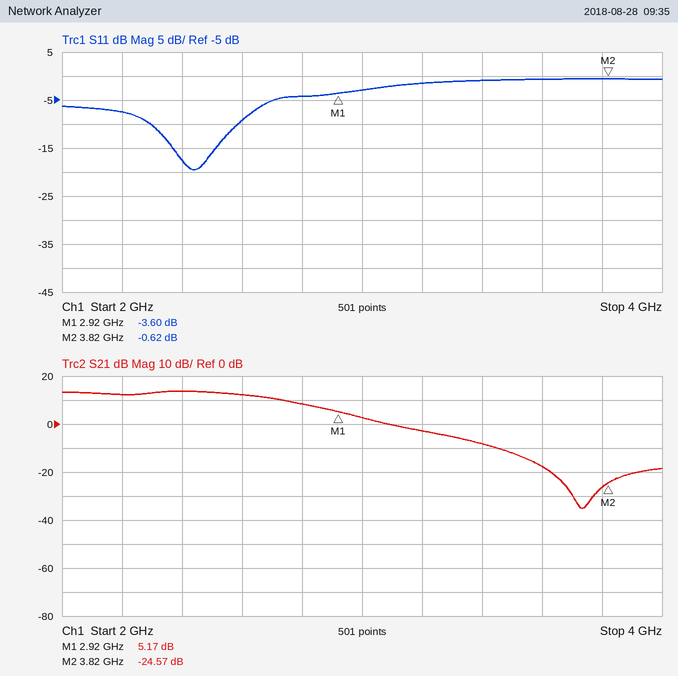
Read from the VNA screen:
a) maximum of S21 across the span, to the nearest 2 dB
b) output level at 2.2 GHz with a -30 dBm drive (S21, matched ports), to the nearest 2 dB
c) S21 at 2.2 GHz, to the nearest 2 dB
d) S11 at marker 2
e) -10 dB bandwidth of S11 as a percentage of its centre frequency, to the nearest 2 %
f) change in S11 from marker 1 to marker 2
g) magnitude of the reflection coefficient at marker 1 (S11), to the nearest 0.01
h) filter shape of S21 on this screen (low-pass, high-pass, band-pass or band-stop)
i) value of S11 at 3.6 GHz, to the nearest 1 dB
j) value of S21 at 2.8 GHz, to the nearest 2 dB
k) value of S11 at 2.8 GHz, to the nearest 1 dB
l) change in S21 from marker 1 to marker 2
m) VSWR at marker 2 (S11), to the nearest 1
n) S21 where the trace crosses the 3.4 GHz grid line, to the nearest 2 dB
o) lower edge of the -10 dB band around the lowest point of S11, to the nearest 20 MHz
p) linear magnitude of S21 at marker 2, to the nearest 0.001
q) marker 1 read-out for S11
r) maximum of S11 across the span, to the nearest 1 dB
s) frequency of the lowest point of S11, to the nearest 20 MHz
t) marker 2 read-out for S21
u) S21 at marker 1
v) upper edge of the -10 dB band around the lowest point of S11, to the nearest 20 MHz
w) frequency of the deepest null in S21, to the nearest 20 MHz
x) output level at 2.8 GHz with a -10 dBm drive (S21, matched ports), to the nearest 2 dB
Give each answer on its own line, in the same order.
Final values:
14 dB
-18 dBm
12 dB
-0.62 dB
12 %
2.98 dB
0.66
low-pass
-1 dB
8 dB
-4 dB
-29.74 dB
28
-8 dB
2.30 GHz
0.059
-3.60 dB
-1 dB
2.44 GHz
-24.57 dB
5.17 dB
2.58 GHz
3.74 GHz
-2 dBm
